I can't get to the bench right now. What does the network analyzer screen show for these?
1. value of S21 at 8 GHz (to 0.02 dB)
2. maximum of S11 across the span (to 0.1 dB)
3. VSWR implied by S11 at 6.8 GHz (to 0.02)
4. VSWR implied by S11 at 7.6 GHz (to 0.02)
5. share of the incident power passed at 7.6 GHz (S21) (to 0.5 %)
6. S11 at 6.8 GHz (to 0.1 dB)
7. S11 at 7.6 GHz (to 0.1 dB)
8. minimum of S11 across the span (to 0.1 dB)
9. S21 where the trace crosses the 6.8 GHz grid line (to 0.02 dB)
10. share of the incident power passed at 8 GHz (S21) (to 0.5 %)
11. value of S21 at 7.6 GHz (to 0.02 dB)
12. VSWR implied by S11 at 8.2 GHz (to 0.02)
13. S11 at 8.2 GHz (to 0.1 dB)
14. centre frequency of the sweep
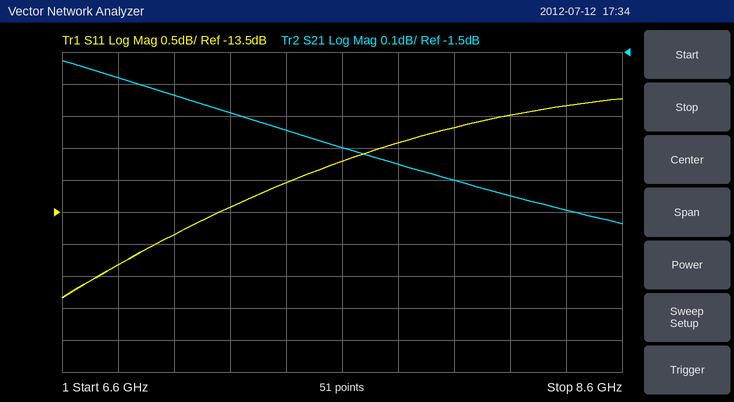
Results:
-1.90 dB
-11.7 dB
1.48
1.60
66.0 %
-14.3 dB
-12.7 dB
-14.8 dB
-1.58 dB
64.5 %
-1.80 dB
1.68
-12.0 dB
7.6 GHz
